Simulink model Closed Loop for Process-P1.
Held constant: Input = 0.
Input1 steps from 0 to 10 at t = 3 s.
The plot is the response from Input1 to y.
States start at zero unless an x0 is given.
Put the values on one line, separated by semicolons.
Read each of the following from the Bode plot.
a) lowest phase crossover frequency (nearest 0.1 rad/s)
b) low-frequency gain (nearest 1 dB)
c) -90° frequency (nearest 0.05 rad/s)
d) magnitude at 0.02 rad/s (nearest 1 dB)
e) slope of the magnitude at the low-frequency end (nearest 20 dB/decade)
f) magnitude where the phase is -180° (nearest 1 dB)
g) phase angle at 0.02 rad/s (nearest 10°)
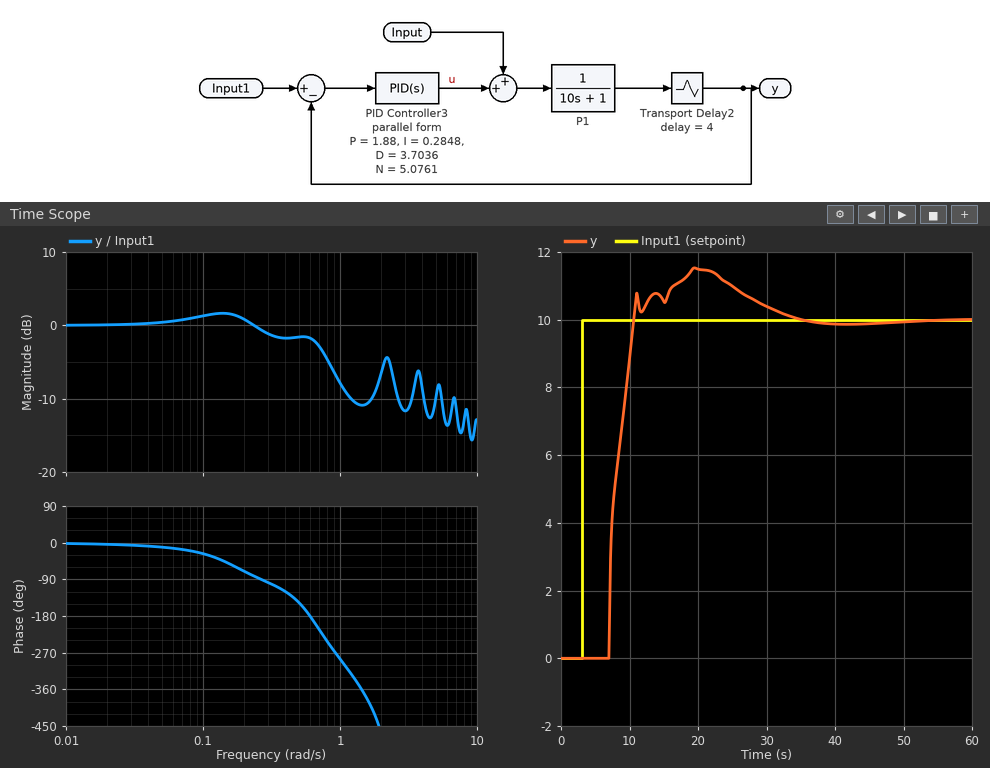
0.6 rad/s; 0 dB; 0.25 rad/s; 0 dB; 0 dB/decade; -2 dB; 0°
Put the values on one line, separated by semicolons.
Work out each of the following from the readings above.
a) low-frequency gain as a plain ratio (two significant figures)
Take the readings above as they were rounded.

1.0
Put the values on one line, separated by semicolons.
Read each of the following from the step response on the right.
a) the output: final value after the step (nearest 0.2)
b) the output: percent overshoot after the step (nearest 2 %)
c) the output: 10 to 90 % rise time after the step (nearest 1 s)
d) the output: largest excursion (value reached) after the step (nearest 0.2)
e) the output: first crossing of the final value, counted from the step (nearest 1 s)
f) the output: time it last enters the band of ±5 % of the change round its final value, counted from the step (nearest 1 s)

10.0; 16 %; 3 s; 11.6; 8 s; 26 s
